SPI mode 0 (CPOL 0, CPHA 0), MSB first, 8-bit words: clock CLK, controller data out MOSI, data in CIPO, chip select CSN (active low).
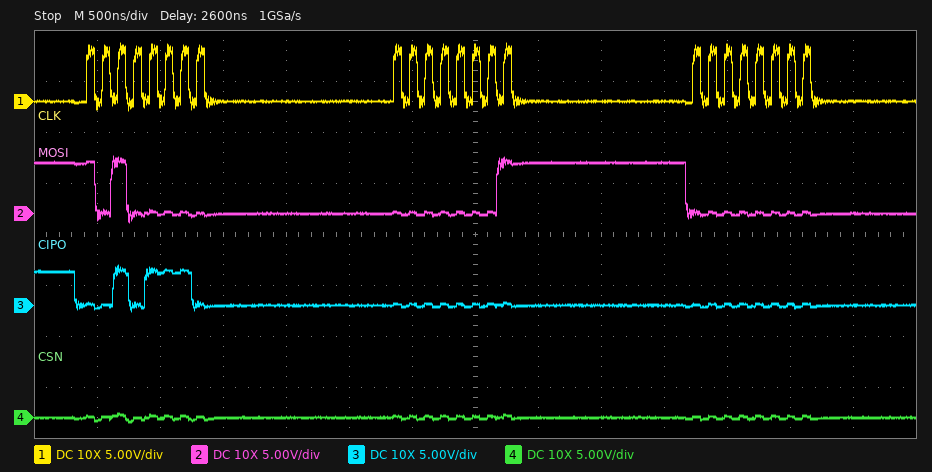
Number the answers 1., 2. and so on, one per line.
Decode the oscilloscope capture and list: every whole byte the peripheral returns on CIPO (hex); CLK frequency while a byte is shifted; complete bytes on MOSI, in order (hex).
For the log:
1. 0x2E 0x00 0x00
2. 8 MHz
3. 0xA0 0x01 0x00
